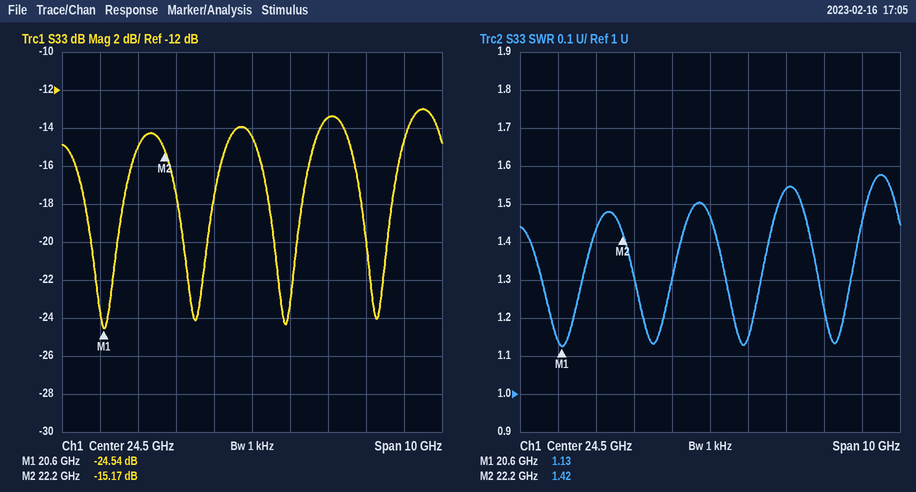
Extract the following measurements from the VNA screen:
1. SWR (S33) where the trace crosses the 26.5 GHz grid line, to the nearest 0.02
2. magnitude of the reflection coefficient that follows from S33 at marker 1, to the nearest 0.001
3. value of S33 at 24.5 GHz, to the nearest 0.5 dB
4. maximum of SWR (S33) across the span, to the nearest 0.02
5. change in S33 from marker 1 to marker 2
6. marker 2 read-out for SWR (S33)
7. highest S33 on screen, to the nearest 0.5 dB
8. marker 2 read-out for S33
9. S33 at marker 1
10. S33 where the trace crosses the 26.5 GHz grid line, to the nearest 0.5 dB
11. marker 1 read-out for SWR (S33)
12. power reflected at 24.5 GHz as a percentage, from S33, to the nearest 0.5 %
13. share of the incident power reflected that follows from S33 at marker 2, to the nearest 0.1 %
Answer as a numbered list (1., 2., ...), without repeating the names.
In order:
1. 1.54
2. 0.059
3. -14.5 dB
4. 1.58
5. 9.37 dB
6. 1.42
7. -13.0 dB
8. -15.17 dB
9. -24.54 dB
10. -13.5 dB
11. 1.13
12. 3.5 %
13. 3.0 %
